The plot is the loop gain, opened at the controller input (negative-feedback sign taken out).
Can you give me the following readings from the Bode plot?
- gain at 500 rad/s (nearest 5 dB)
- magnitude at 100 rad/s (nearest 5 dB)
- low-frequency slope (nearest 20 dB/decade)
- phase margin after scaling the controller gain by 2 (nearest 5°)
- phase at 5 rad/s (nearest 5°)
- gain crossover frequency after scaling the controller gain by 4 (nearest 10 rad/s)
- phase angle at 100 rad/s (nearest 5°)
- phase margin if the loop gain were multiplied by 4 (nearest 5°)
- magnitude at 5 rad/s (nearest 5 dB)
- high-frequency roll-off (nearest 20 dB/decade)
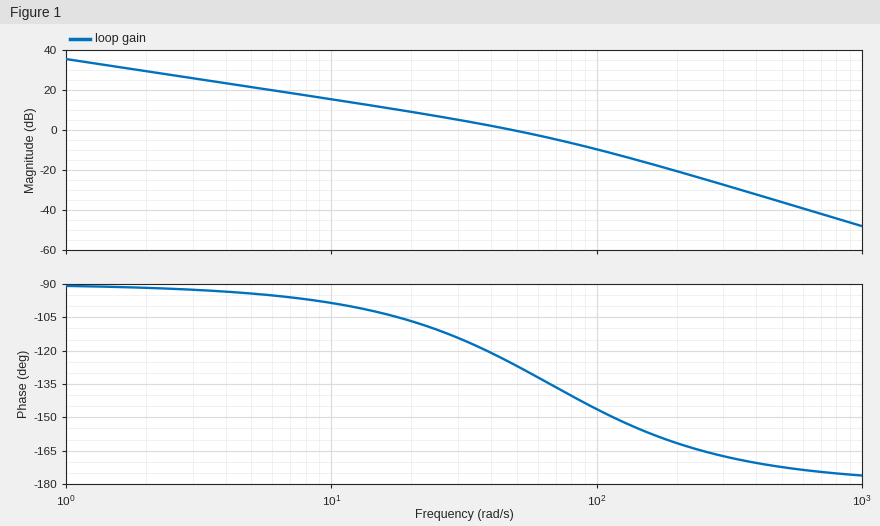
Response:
-35 dB
-10 dB
-20 dB/decade
40°
-95°
120 rad/s
-145°
30°
20 dB
-40 dB/decade
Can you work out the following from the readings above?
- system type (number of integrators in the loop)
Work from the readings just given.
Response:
1
